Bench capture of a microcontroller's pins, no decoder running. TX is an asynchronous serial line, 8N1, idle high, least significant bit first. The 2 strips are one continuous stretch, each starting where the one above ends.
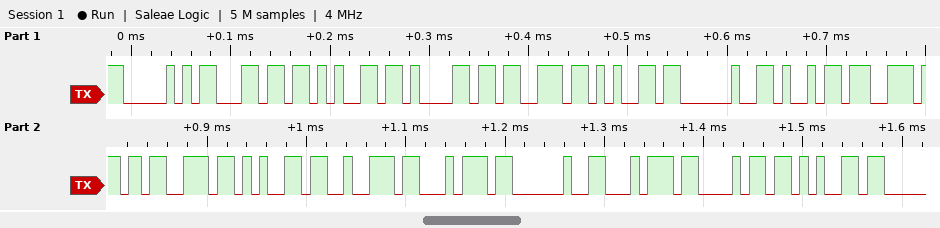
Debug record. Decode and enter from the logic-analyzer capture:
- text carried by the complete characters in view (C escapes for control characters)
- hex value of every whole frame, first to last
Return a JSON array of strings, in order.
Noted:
["\"Please insert the\"", "50 6C 65 61 73 65 20 69 6E 73 65 72 74 20 74 68 65"]
